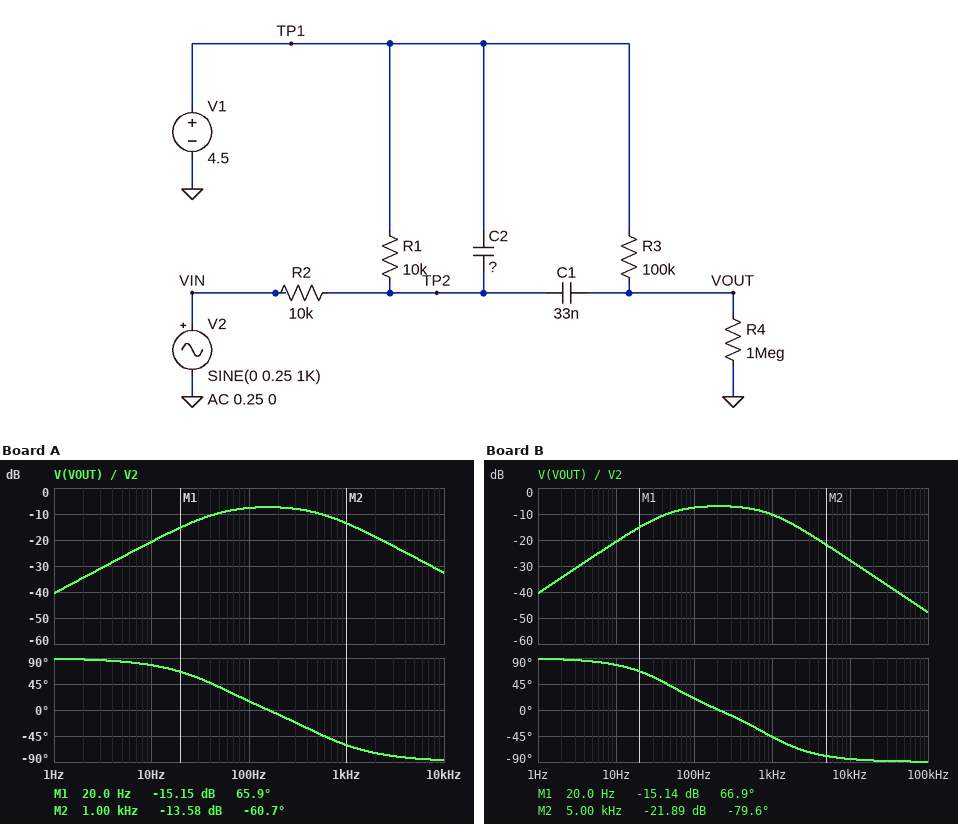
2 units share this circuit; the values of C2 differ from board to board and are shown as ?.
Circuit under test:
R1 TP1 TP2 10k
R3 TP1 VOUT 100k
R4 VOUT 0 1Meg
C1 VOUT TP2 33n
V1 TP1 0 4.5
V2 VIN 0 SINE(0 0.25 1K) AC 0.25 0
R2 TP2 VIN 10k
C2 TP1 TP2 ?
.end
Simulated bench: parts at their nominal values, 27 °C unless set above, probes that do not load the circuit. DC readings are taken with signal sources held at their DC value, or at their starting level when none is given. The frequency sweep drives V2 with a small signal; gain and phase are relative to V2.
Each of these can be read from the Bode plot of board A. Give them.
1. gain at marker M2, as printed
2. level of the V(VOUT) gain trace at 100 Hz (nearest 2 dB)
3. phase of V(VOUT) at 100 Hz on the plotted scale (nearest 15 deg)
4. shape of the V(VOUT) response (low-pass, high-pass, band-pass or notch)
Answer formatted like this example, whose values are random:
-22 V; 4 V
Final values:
-13.58 dB; -8 dB; 15 deg; band-pass
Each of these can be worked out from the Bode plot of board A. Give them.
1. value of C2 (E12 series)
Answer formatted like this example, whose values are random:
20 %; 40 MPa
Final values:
68 nF
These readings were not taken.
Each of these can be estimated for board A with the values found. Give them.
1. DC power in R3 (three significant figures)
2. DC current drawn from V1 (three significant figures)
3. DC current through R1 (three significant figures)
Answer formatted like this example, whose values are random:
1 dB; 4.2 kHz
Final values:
1.67 µW; 229 µA; 225 µA
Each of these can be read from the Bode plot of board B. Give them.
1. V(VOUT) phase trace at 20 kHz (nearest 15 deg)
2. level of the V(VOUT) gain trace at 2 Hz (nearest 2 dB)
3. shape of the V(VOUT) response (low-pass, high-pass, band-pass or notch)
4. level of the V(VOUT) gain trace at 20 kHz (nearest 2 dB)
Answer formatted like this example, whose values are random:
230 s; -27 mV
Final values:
-90 deg; -34 dB; band-pass; -34 dB
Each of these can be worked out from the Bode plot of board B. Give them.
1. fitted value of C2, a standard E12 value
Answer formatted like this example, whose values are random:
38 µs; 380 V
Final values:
39 nF
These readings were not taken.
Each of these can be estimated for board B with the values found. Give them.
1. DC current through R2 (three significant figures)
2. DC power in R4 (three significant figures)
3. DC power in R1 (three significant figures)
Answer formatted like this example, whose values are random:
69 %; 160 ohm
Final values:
225 µA; 16.7 µW; 506 µW
